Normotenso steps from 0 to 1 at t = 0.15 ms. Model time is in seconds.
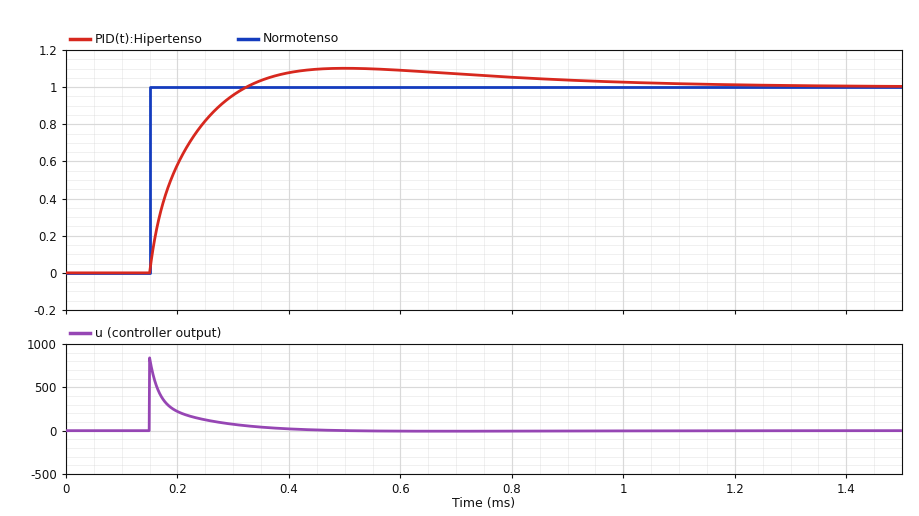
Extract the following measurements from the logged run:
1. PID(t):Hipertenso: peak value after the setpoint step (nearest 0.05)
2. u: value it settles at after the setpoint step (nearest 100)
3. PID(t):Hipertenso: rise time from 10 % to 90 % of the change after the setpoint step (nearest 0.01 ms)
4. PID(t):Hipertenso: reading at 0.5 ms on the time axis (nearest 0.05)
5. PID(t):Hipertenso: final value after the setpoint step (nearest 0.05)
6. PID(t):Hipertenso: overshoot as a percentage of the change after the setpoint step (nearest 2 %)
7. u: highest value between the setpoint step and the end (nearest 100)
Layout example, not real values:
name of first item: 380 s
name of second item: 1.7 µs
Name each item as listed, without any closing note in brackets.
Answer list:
PID(t):Hipertenso: peak value after the setpoint step: 1.10
u: value it settles at after the setpoint step: 0
PID(t):Hipertenso: rise time from 10 % to 90 % of the change after the setpoint step: 0.12 ms
PID(t):Hipertenso: reading at 0.5 ms on the time axis: 1.10
PID(t):Hipertenso: final value after the setpoint step: 1.00
PID(t):Hipertenso: overshoot as a percentage of the change after the setpoint step: 10 %
u: highest value between the setpoint step and the end: 800
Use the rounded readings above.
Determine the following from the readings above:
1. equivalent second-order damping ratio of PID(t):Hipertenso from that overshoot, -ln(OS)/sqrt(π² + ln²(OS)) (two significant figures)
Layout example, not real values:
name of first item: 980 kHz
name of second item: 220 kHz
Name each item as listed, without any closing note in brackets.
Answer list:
equivalent second-order damping ratio of PID(t):Hipertenso from that overshoot, -ln(OS)/sqrt(π² + ln²(OS)): 0.59
